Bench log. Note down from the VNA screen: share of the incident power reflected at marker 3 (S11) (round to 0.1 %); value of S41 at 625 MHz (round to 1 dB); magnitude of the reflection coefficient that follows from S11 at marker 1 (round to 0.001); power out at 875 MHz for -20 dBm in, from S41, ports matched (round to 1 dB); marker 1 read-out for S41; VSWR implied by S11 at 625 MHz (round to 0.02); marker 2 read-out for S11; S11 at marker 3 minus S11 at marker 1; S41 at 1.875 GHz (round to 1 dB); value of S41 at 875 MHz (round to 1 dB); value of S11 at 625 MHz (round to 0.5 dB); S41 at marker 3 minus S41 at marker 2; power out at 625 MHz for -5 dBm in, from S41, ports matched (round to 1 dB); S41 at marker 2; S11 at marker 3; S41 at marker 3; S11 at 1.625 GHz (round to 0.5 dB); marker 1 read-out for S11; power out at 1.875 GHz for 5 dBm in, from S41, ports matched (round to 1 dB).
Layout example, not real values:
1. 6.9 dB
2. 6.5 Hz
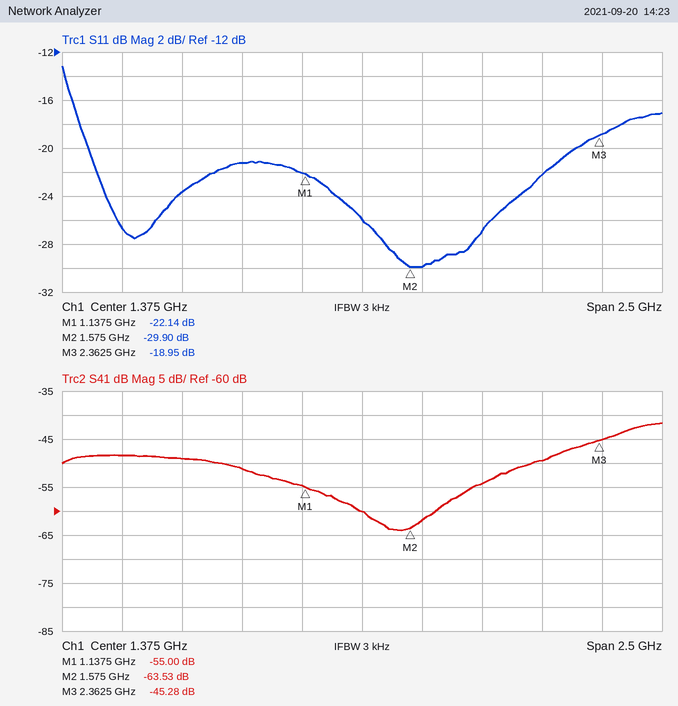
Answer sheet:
1. 1.3 %
2. -49 dB
3. 0.078
4. -71 dBm
5. -55.00 dB
6. 1.14
7. -29.90 dB
8. 3.19 dB
9. -54 dB
10. -51 dB
11. -23.5 dB
12. 18.25 dB
13. -54 dBm
14. -63.53 dB
15. -18.95 dB
16. -45.28 dB
17. -30.0 dB
18. -22.14 dB
19. -49 dBm
